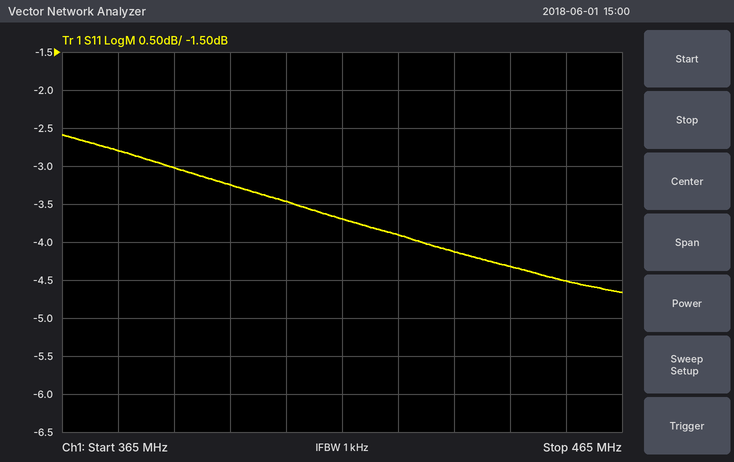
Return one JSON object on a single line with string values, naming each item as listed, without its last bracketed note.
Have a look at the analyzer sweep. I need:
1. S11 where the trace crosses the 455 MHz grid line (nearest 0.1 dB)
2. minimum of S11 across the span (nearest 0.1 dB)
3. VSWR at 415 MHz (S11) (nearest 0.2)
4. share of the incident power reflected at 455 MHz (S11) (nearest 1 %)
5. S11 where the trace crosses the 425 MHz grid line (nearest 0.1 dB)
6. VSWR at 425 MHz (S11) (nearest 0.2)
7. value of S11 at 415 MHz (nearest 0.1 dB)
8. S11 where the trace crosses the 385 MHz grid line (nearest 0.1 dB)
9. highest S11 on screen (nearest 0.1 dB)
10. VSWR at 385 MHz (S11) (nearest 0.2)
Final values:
{"S11 where the trace crosses the 455 MHz grid line": "-4.5 dB", "minimum of S11 across the span": "-4.7 dB", "VSWR at 415 MHz (S11)": "4.8", "share of the incident power reflected at 455 MHz (S11)": "35 %", "S11 where the trace crosses the 425 MHz grid line": "-3.9 dB", "VSWR at 425 MHz (S11)": "4.6", "value of S11 at 415 MHz": "-3.7 dB", "S11 where the trace crosses the 385 MHz grid line": "-3.0 dB", "highest S11 on screen": "-2.6 dB", "VSWR at 385 MHz (S11)": "5.8"}
